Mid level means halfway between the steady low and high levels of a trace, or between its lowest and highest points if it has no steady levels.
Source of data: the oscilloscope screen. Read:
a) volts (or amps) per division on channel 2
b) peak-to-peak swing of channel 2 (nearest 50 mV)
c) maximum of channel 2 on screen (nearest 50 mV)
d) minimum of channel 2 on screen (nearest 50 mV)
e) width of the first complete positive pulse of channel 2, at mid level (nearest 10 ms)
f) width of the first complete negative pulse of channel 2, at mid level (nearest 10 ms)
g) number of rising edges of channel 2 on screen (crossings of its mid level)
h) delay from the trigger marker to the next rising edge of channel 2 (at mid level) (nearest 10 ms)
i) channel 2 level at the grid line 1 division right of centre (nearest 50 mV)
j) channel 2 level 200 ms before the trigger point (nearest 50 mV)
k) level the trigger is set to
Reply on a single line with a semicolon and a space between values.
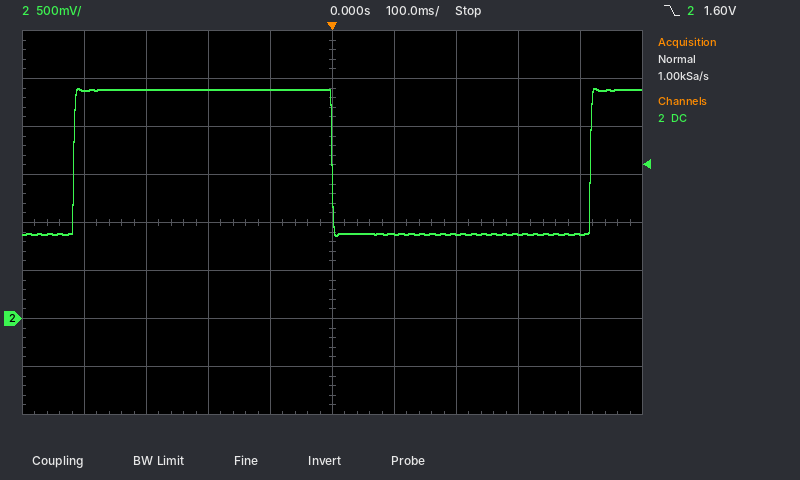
500 mV; 1.55 V; 2.40 V; 850 mV; 420 ms; 420 ms; 2; 420 ms; 900 mV; 2.40 V; 1.60 V
